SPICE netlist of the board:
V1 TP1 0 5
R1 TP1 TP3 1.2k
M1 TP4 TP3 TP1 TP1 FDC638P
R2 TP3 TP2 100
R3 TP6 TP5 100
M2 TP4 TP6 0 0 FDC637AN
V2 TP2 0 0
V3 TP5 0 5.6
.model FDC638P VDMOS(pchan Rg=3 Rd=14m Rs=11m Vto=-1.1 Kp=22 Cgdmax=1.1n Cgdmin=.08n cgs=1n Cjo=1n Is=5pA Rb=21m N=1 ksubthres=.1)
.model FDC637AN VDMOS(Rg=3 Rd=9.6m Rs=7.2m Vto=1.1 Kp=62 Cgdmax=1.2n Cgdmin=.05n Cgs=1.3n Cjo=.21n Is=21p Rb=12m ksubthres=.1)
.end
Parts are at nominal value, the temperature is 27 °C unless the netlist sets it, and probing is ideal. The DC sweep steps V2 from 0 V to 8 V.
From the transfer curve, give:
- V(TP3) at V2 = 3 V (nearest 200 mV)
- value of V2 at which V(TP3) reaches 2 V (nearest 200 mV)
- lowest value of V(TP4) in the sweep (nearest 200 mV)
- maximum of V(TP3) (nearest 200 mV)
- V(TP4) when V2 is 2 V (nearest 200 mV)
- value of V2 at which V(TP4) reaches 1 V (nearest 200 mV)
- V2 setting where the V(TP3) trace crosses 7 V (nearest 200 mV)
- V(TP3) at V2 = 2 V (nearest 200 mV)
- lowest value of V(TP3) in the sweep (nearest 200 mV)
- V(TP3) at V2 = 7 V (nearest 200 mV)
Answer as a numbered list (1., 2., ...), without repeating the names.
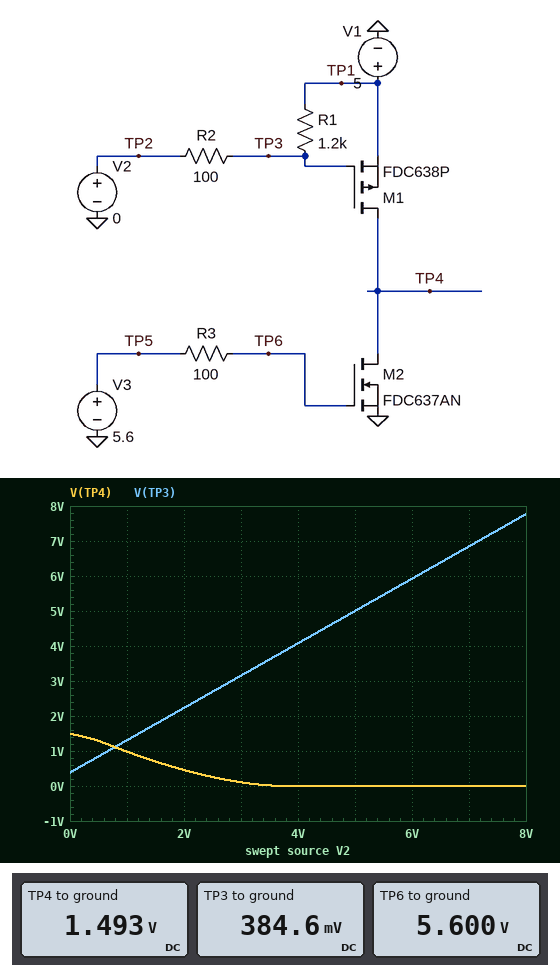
1. 3.2 V
2. 1.8 V
3. 0 V
4. 7.8 V
5. 400 mV
6. 1.0 V
7. 7.2 V
8. 2.2 V
9. 400 mV
10. 6.8 V
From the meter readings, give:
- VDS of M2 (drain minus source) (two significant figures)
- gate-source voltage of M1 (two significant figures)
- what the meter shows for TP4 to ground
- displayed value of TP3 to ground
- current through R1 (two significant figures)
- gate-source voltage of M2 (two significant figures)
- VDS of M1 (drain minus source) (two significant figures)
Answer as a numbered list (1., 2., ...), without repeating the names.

1. 1.5 V
2. -4.6 V
3. 1.493 V
4. 384.6 mV
5. 3.8 mA
6. 5.6 V
7. -3.5 V
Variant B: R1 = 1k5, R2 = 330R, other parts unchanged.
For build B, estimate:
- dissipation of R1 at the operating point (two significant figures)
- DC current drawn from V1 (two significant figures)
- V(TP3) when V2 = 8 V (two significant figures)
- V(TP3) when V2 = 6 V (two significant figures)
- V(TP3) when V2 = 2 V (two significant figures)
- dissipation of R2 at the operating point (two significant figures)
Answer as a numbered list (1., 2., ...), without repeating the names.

1. 11 mW
2. 60 A
3. 7.5 V
4. 5.8 V
5. 2.5 V
6. 2.5 mW
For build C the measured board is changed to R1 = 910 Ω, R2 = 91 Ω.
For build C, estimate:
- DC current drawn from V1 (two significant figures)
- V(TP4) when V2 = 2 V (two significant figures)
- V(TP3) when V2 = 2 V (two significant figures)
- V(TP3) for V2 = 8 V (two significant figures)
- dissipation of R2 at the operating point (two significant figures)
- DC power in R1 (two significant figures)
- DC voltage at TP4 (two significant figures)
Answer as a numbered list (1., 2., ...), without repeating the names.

1. 70 A
2. 440 mV
3. 2.3 V
4. 7.7 V
5. 2.3 mW
6. 23 mW
7. 1.5 V
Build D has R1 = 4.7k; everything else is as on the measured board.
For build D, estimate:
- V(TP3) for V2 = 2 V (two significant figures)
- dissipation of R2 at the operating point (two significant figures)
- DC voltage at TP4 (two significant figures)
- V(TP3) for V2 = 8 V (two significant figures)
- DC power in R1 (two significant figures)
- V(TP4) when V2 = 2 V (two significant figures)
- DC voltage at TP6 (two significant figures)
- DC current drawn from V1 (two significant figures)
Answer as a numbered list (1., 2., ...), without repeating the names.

1. 2.1 V
2. 110 µW
3. 1.6 V
4. 7.9 V
5. 5.1 mW
6. 540 mV
7. 5.6 V
8. 75 A
